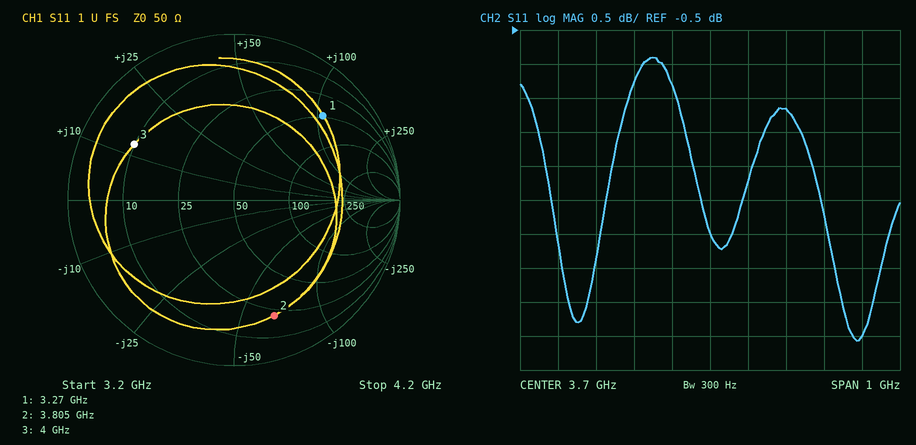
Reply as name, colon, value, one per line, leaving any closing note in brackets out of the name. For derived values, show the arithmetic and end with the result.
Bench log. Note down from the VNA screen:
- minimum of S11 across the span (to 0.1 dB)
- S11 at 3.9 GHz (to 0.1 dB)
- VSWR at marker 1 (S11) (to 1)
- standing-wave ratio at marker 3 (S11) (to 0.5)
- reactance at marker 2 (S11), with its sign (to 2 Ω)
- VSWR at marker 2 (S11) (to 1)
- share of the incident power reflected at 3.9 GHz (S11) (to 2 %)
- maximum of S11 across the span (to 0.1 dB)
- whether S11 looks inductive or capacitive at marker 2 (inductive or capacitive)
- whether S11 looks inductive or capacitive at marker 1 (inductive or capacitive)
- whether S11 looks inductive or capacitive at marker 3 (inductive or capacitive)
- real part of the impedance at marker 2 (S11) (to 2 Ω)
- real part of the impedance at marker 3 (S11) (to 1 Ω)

minimum of S11 across the span: -5.1 dB
S11 at 3.9 GHz: -1.7 dB
VSWR at marker 1 (S11): 7
standing-wave ratio at marker 3 (S11): 5.5
reactance at marker 2 (S11), with its sign: -66 Ω
VSWR at marker 2 (S11): 7
share of the incident power reflected at 3.9 GHz (S11): 10^(-1.7/10) ≈ 68 %
maximum of S11 across the span: -0.9 dB
whether S11 looks inductive or capacitive at marker 2: capacitive
whether S11 looks inductive or capacitive at marker 1: inductive
whether S11 looks inductive or capacitive at marker 3: inductive
real part of the impedance at marker 2 (S11): 22 Ω
real part of the impedance at marker 3 (S11): 10 Ω
